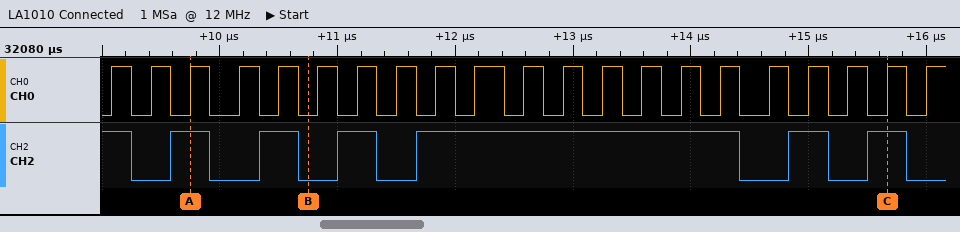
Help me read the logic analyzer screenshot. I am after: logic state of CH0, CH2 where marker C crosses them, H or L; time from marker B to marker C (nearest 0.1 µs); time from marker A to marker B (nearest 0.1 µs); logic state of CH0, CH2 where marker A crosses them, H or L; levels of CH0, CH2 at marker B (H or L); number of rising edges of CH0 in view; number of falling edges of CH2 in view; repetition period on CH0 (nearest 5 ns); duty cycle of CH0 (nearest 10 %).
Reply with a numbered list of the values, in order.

1. CH0=H, CH2=H
2. 4.9 µs
3. 1 µs
4. CH0=H, CH2=H
5. CH0=L, CH2=L
6. 21
7. 7
8. 345 ns
9. 50 %
